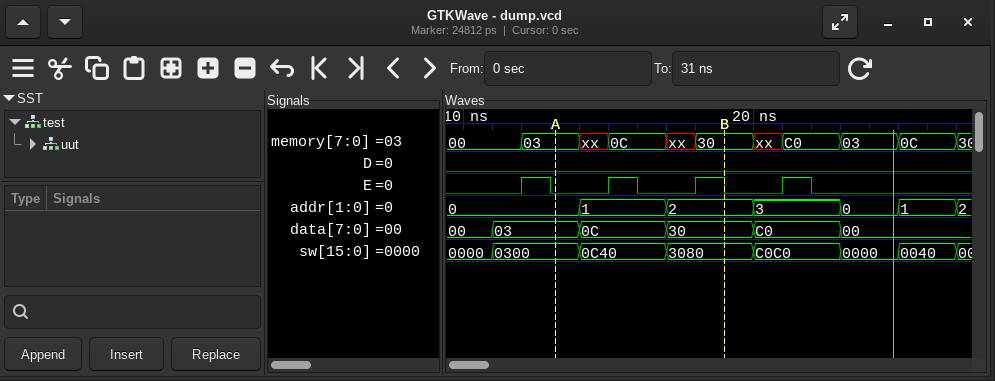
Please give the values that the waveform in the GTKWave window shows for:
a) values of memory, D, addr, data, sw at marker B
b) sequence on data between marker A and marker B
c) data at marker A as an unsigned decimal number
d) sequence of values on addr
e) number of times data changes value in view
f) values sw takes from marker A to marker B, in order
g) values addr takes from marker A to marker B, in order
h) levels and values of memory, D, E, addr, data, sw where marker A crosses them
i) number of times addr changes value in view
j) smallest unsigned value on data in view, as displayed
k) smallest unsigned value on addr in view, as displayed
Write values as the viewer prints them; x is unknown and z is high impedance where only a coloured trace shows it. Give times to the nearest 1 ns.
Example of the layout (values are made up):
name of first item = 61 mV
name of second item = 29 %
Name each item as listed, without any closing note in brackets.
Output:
values of memory, D, addr, data, sw at marker B = memory=30, D=0, addr=2, data=30, sw=3080
sequence on data between marker A and marker B = 03, 0C, 30
data at marker A as an unsigned decimal number = 3
sequence of values on addr = 0, 1, 2, 3, 0, 1, 2
number of times data changes value in view = 5
values sw takes from marker A to marker B, in order = 0300, 0C40, 3080
values addr takes from marker A to marker B, in order = 0, 1, 2
levels and values of memory, D, E, addr, data, sw where marker A crosses them = memory=03, D=0, E=0, addr=0, data=03, sw=0300
number of times addr changes value in view = 6
smallest unsigned value on data in view, as displayed = 00
smallest unsigned value on addr in view, as displayed = 0
